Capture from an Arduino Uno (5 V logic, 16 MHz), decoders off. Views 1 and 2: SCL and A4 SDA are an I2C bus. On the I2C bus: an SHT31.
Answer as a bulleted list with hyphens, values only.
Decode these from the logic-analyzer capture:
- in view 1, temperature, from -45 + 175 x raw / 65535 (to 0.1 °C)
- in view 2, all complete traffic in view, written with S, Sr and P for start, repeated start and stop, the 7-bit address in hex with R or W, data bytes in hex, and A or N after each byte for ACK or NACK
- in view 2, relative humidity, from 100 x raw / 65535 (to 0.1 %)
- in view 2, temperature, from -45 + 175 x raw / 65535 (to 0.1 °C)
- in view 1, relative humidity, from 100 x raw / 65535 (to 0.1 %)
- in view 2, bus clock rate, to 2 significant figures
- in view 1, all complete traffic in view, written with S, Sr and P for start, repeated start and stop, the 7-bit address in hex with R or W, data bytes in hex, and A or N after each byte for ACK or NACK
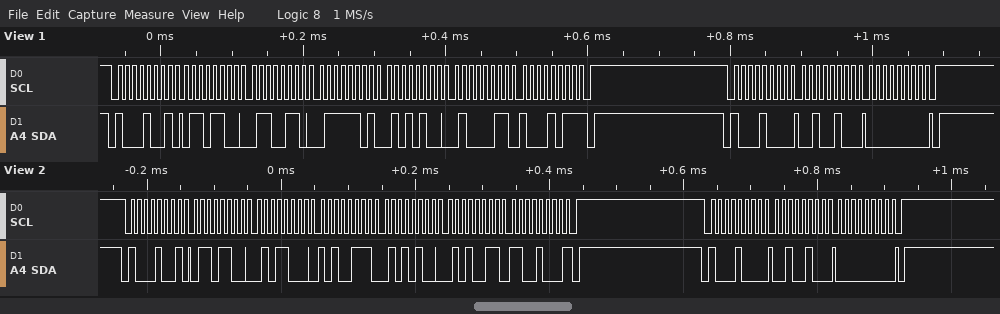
- 29.1 °C
- S 44R A 6C A 58 A A7 A 54 A 53 A C8 N P S 44W A 24 A 00 A P
- 32.9 %
- 29.1 °C
- 32.9 %
- 100 kHz
- S 44R A 6C A 66 A 7D A 54 A 43 A 8B N P S 44W A 24 A 00 A P
